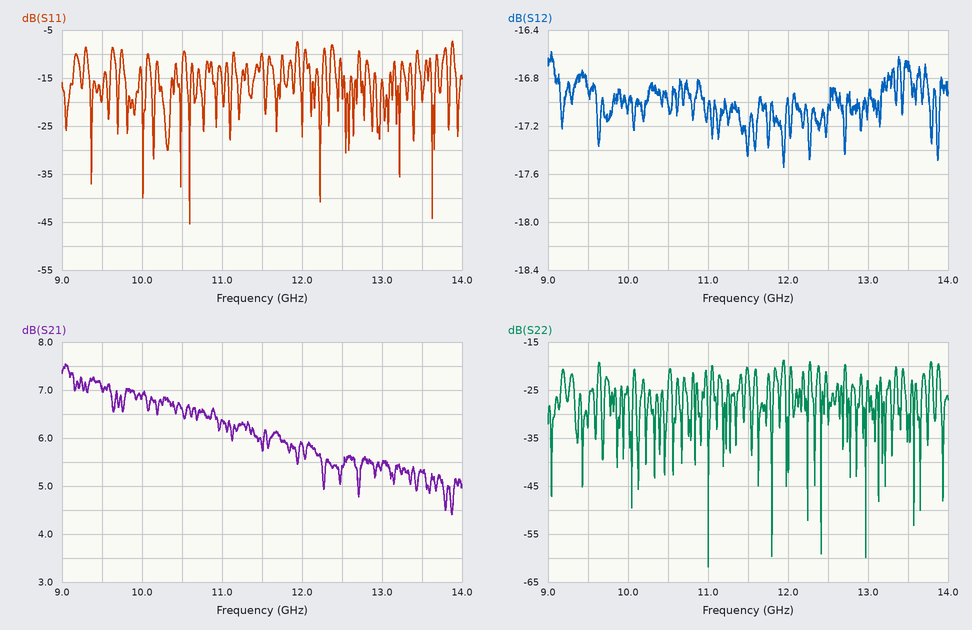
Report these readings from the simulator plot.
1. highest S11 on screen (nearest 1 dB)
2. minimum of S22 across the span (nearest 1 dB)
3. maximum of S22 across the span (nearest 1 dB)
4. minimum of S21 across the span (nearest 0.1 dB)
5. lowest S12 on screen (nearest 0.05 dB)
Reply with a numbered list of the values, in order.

1. -7 dB
2. -62 dB
3. -19 dB
4. 4.4 dB
5. -17.55 dB
